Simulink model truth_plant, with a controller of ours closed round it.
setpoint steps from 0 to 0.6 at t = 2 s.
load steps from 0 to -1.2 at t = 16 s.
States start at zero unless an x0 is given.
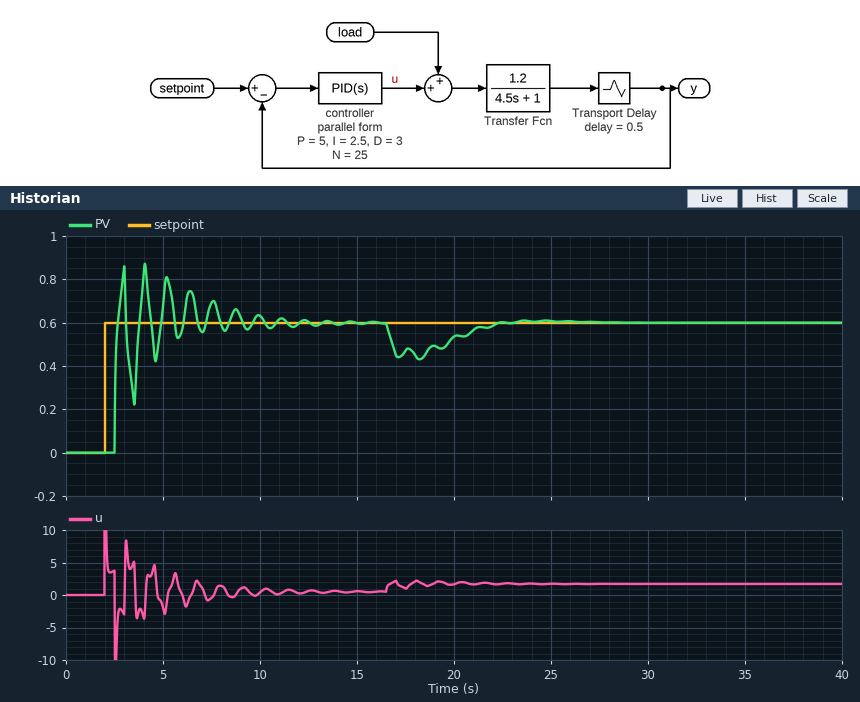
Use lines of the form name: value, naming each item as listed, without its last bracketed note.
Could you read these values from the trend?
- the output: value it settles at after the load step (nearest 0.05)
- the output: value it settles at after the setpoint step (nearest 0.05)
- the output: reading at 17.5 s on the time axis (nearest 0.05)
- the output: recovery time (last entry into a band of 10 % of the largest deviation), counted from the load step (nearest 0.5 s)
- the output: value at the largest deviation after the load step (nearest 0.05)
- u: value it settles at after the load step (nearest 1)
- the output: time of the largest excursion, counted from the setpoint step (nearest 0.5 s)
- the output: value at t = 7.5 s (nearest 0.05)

the output: value it settles at after the load step: 0.60
the output: value it settles at after the setpoint step: 0.60
the output: reading at 17.5 s on the time axis: 0.45
the output: recovery time (last entry into a band of 10 % of the largest deviation), counted from the load step: 6.0 s
the output: value at the largest deviation after the load step: 0.45
u: value it settles at after the load step: 2
the output: time of the largest excursion, counted from the setpoint step: 2.0 s
the output: value at t = 7.5 s: 0.70
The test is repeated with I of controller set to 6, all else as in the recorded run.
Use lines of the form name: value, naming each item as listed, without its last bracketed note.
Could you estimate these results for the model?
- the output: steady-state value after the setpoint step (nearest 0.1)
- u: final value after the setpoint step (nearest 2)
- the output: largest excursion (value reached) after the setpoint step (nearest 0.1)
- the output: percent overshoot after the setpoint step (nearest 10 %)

the output: steady-state value after the setpoint step: 0.6
u: final value after the setpoint step: 0
the output: largest excursion (value reached) after the setpoint step: 1.0
the output: percent overshoot after the setpoint step: 60 %
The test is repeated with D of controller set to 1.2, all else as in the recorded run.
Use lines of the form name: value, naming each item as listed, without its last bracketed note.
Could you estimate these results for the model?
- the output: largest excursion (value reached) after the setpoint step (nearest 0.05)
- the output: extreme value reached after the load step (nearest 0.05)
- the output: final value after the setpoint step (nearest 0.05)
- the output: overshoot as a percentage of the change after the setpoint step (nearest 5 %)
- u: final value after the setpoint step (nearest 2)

the output: largest excursion (value reached) after the setpoint step: 0.70
the output: extreme value reached after the load step: 0.40
the output: final value after the setpoint step: 0.60
the output: overshoot as a percentage of the change after the setpoint step: 15 %
u: final value after the setpoint step: 0
